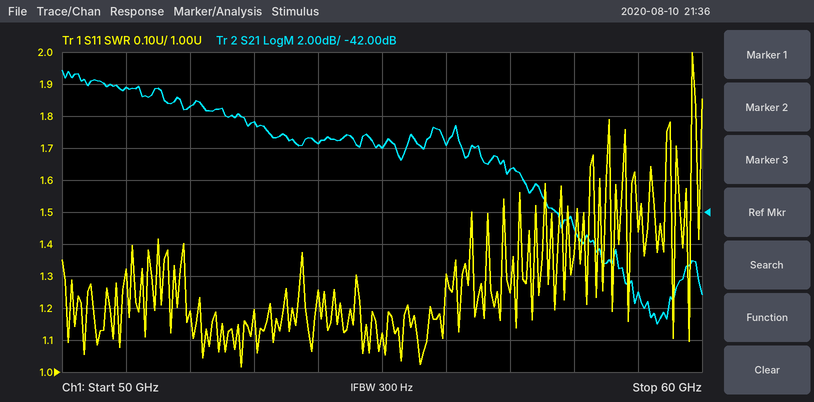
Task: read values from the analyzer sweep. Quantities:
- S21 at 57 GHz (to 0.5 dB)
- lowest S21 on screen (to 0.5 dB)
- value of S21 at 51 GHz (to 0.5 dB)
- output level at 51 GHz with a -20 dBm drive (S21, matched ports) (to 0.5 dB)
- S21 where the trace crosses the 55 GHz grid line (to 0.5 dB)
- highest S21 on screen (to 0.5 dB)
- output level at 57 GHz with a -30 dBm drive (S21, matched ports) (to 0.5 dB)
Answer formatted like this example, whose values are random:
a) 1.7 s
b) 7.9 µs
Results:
a) -39.5 dB
b) -49.0 dB
c) -34.0 dB
d) -54.0 dBm
e) -38.0 dB
f) -33.0 dB
g) -69.5 dBm
